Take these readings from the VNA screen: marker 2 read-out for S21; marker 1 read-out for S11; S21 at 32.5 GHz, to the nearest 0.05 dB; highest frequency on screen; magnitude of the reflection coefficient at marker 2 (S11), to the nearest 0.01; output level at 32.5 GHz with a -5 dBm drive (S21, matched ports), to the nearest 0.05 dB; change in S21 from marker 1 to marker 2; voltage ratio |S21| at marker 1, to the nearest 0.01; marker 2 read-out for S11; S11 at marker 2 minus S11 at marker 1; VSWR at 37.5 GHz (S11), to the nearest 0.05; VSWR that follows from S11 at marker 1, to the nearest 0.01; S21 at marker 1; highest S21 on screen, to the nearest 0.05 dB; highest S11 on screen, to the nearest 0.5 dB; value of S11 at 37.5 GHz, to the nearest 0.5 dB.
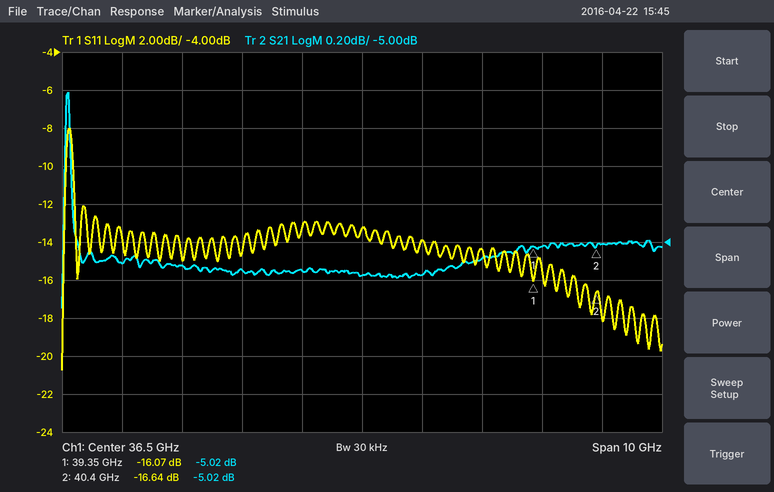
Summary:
-5.02 dB
-16.07 dB
-5.10 dB
41.5 GHz
0.15
-10.10 dBm
0.00 dB
0.56
-16.64 dB
-0.57 dB
1.50
1.37
-5.02 dB
-4.20 dB
-8.0 dB
-14.0 dB
